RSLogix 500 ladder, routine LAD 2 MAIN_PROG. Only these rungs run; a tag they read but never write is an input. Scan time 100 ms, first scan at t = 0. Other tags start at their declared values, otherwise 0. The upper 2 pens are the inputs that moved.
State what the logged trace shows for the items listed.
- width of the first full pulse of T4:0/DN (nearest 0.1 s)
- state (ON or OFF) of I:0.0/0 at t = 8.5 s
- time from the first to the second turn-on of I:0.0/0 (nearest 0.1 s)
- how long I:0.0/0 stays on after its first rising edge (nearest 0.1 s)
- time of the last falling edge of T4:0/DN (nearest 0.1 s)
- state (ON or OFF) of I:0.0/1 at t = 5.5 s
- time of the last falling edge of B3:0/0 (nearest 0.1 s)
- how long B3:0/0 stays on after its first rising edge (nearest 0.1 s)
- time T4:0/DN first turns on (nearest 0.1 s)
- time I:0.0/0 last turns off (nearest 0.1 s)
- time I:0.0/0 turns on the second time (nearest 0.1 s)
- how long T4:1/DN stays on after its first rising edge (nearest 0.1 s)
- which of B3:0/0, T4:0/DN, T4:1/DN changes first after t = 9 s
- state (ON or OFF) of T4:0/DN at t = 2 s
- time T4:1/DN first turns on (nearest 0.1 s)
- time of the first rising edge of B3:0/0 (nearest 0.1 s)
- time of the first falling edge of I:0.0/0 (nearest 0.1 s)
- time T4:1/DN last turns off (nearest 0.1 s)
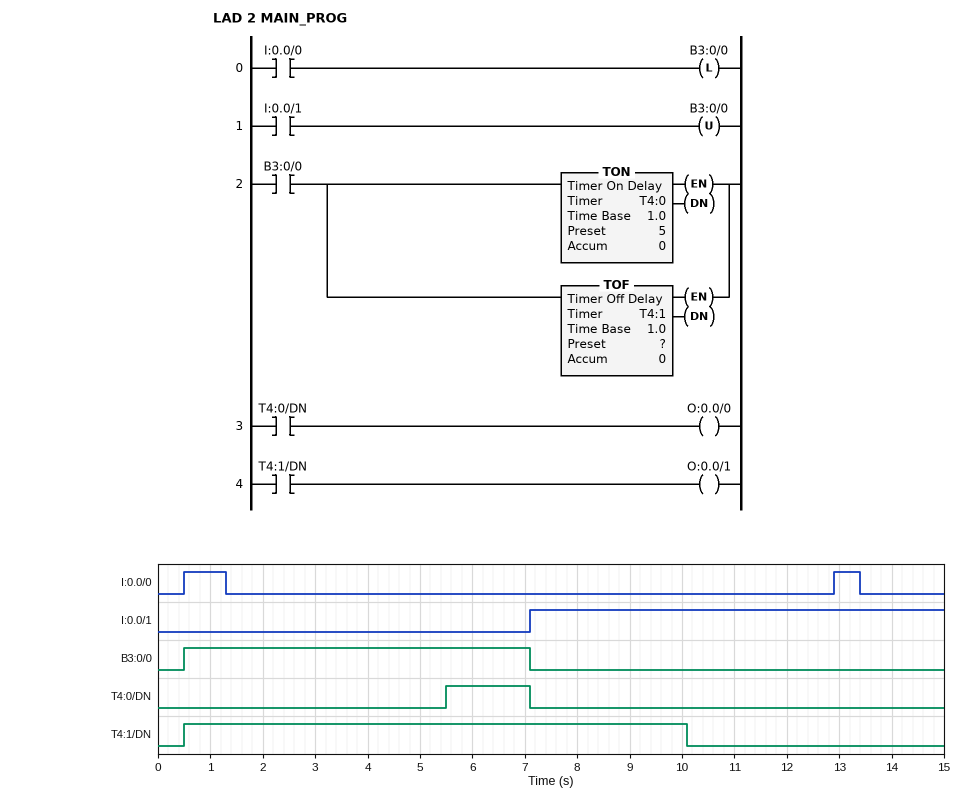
1.6 s
OFF
12.4 s
0.8 s
7.1 s
OFF
7.1 s
6.6 s
5.5 s
13.4 s
12.9 s
9.6 s
T4:1/DN
OFF
0.5 s
0.5 s
1.3 s
10.1 s
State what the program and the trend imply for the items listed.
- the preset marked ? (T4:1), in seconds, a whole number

3 s
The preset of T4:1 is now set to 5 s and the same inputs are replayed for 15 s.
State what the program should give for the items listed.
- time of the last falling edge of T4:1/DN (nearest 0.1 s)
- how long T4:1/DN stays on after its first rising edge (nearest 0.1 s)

12.1 s
11.6 s
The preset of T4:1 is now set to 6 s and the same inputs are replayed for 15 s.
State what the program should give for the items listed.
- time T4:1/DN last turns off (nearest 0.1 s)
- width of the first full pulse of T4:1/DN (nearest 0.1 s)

13.1 s
12.6 s
